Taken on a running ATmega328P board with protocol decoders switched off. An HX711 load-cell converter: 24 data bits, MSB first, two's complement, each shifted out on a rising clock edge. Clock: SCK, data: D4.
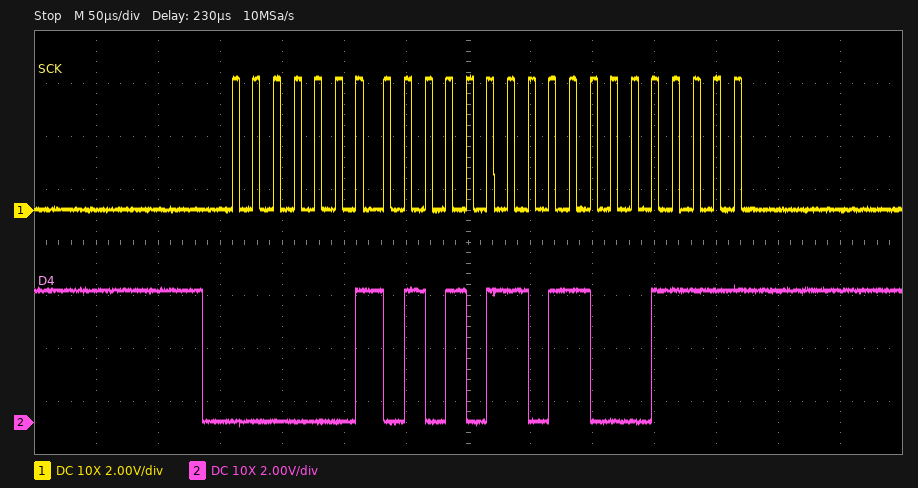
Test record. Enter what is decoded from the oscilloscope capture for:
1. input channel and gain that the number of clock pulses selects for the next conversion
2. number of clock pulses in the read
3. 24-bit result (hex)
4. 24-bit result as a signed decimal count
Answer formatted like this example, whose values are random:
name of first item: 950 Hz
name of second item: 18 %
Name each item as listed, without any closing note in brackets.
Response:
input channel and gain that the number of clock pulses selects for the next conversion: channel A, gain 128
number of clock pulses in the read: 25
24-bit result: 0x02AD8F
24-bit result as a signed decimal count: 175503
